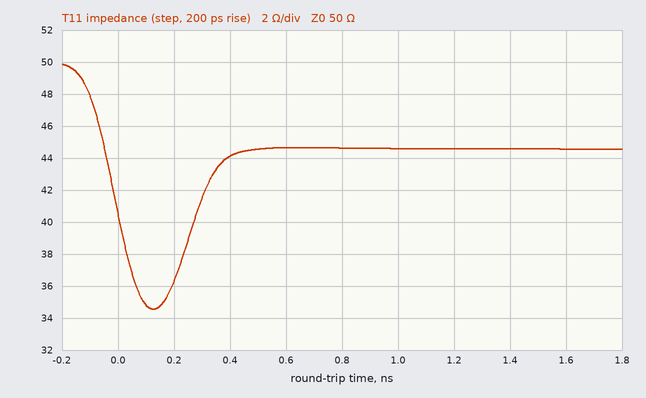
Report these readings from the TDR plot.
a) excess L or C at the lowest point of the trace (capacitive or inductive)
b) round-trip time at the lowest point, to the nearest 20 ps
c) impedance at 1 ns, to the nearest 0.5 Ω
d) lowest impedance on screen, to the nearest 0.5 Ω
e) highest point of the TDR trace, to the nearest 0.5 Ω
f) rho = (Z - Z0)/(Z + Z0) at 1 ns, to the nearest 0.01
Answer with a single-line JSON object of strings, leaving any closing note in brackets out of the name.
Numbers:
{"excess L or C at the lowest point of the trace": "capacitive", "round-trip time at the lowest point, to the nearest 20 ps": "120 ps", "impedance at 1 ns, to the nearest 0.5 Ω": "44.5 Ω", "lowest impedance on screen, to the nearest 0.5 Ω": "34.5 Ω", "highest point of the TDR trace, to the nearest 0.5 Ω": "50.0 Ω", "rho = (Z - Z0)/(Z + Z0) at 1 ns, to the nearest 0.01": "-0.06"}
